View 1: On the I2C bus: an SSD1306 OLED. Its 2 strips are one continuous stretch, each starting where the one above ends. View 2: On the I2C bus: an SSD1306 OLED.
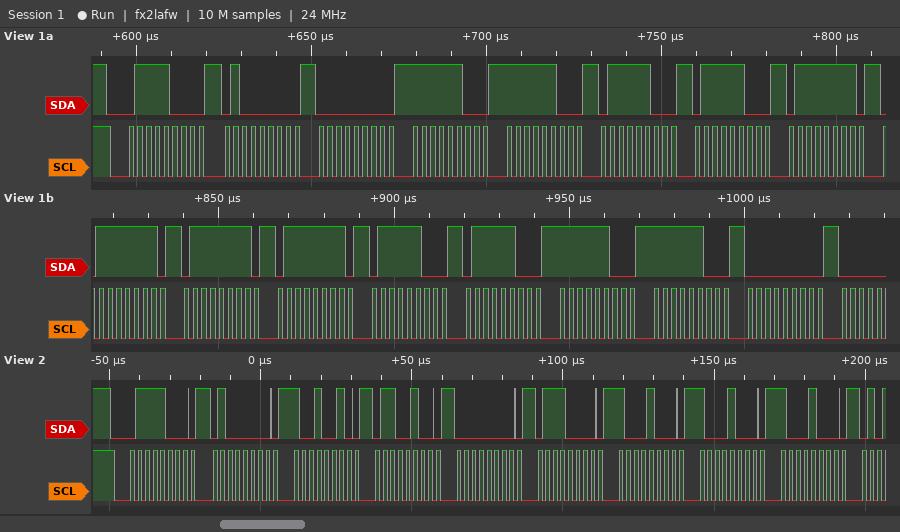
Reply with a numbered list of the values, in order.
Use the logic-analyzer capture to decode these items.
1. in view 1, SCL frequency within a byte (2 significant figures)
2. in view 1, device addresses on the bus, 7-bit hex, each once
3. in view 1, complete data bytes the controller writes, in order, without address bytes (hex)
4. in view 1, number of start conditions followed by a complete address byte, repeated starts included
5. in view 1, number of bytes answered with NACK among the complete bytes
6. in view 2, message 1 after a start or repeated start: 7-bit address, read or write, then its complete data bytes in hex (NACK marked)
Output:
1. 400 kHz
2. 0x3C
3. 40 00 FC FC 7C 7C 7F 7F 7F 7F 7C 7C FC FC 00
4. 1
5. 0
6. 0x3C write: 40 92 64 00 70 88 88 88
